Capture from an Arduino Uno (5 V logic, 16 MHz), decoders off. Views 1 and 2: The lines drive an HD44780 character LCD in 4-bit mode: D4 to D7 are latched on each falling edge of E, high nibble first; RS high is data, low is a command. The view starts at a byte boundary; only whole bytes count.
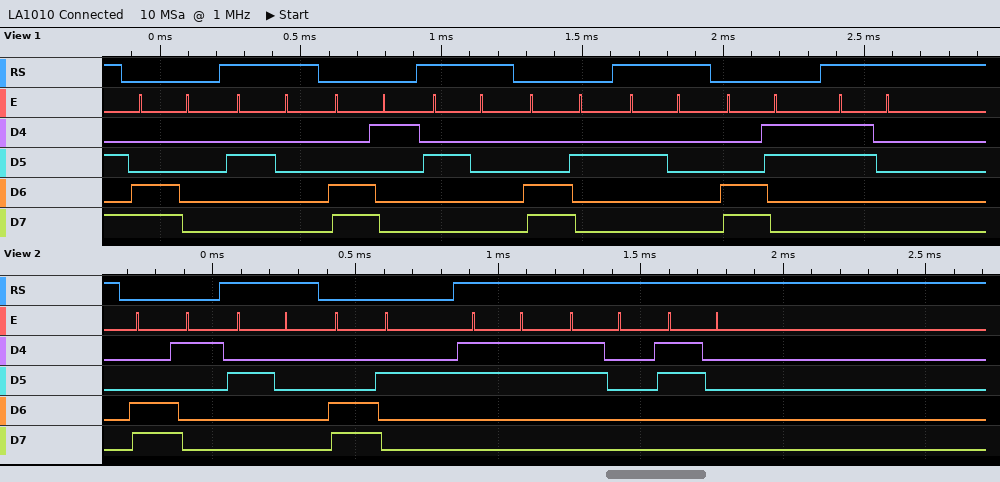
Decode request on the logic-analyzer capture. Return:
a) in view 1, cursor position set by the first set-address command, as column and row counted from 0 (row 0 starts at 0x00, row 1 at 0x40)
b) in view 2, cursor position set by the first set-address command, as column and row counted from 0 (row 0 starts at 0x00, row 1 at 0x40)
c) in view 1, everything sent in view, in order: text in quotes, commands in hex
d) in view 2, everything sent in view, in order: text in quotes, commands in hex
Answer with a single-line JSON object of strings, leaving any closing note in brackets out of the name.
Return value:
{"in view 1, cursor position set by the first set-address command, as column and row counted from 0": "column 0, row 1", "in view 2, cursor position set by the first set-address command, as column and row counted from 0": "column 1, row 1", "in view 1, everything sent in view, in order: text in quotes, commands in hex": "0xC0 \" \" 0xC1 \" \" 0xC2 \" \" 0xC3 \"0\"", "in view 2, everything sent in view, in order: text in quotes, commands in hex": "0xC1 \" \" 0xC2 \"300\""}
